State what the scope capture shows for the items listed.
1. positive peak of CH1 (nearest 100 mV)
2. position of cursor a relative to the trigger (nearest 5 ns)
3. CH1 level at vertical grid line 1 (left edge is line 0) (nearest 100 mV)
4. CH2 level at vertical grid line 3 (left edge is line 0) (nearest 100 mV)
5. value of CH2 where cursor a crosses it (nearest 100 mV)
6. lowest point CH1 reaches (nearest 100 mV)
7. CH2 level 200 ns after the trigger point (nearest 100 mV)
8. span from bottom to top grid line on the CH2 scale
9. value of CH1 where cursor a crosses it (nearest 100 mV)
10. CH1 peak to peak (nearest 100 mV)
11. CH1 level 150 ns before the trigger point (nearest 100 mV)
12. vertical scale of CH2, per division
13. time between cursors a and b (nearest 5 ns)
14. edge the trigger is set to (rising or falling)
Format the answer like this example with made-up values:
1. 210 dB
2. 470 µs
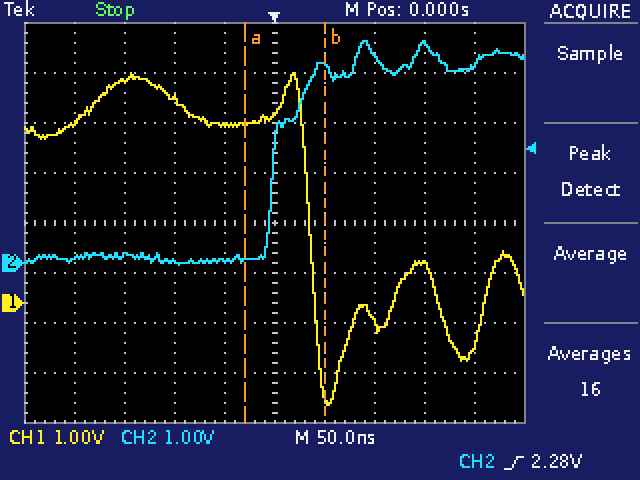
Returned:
1. 4.6 V
2. -30 ns
3. 3.6 V
4. 0.0 V
5. 100 mV
6. -2.0 V
7. 4.0 V
8. 8 V
9. 3.6 V
10. 6.6 V
11. 4.4 V
12. 1 V
13. 80 ns
14. rising
